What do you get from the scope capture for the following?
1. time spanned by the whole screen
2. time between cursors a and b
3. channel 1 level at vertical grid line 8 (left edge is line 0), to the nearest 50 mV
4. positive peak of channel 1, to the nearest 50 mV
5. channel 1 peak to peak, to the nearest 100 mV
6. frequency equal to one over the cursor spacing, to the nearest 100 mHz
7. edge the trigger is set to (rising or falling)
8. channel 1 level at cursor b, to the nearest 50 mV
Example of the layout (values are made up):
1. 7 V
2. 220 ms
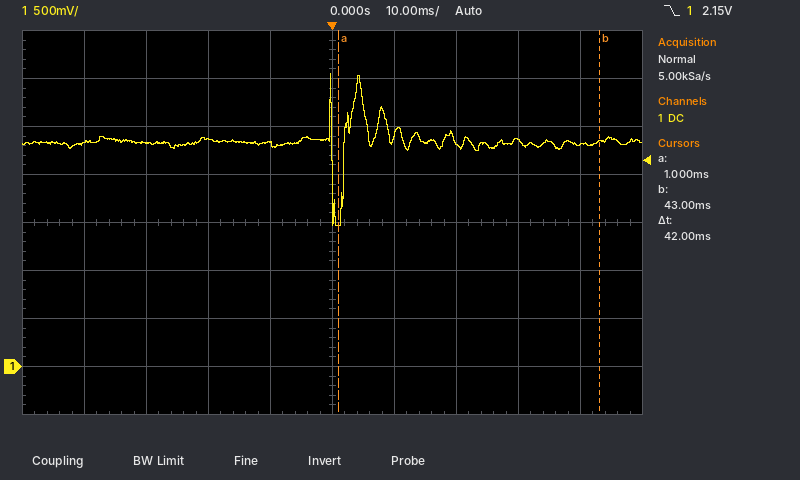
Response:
1. 100 ms
2. 42 ms
3. 2.35 V
4. 3.05 V
5. 1.60 V
6. 23.8 Hz
7. falling
8. 2.35 V
